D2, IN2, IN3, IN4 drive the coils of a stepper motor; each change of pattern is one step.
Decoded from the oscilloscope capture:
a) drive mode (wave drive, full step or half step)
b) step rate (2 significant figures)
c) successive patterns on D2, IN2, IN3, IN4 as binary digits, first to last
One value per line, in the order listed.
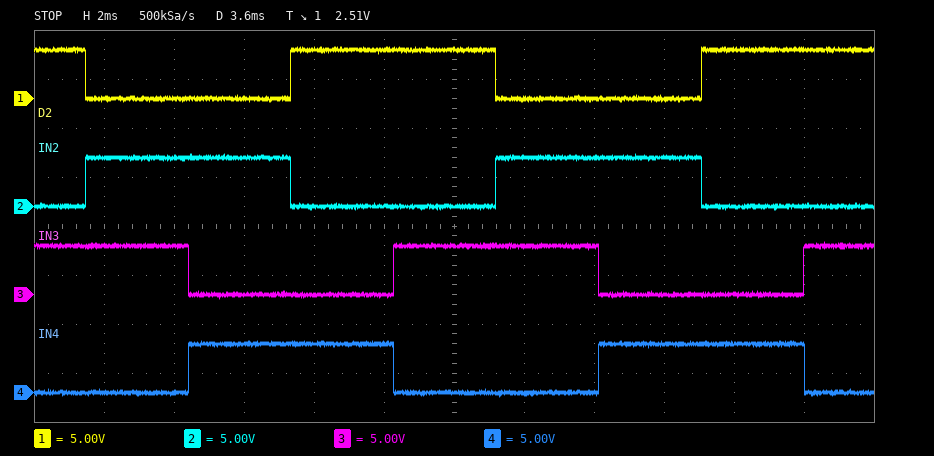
full step
340 steps/s
1010 0110 0101 1001 1010 0110 0101 1001 1010
